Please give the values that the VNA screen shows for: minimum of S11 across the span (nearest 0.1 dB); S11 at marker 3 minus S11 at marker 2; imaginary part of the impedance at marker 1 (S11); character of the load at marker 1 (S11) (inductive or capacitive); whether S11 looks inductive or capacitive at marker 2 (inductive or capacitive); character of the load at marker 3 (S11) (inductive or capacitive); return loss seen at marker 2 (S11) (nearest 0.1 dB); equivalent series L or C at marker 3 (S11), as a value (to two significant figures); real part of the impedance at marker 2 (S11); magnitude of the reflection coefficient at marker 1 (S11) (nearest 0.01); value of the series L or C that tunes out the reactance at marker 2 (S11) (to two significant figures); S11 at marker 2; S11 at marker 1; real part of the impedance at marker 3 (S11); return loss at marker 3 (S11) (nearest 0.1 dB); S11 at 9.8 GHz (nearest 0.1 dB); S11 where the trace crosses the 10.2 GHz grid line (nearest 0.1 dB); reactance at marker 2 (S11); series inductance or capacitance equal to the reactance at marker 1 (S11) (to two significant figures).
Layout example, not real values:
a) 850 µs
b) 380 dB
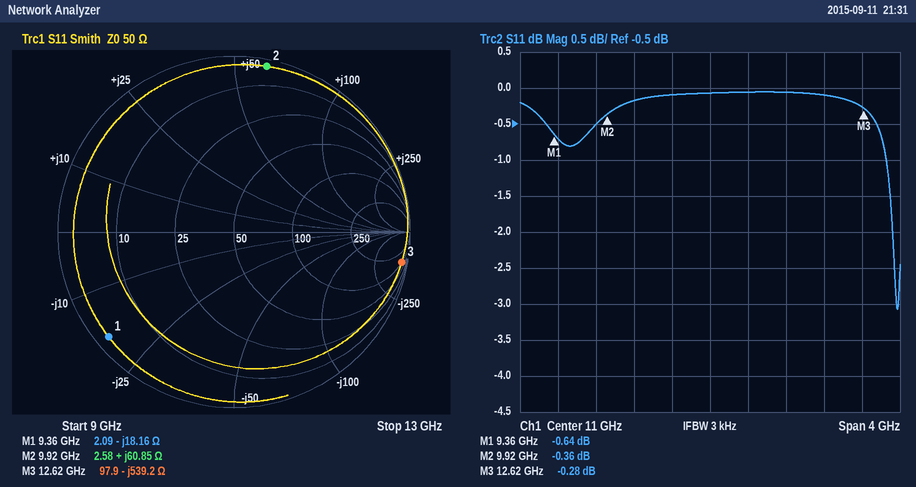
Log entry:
a) -3.1 dB
b) 0.08 dB
c) -18.16 Ω
d) capacitive
e) inductive
f) capacitive
g) 0.4 dB
h) 23 fF
i) 2.58 Ω
j) 0.93
k) 260 fF
l) -0.36 dB
m) -0.64 dB
n) 97.9 Ω
o) 0.3 dB
p) -0.5 dB
q) -0.2 dB
r) +60.85 Ω
s) 940 fF
